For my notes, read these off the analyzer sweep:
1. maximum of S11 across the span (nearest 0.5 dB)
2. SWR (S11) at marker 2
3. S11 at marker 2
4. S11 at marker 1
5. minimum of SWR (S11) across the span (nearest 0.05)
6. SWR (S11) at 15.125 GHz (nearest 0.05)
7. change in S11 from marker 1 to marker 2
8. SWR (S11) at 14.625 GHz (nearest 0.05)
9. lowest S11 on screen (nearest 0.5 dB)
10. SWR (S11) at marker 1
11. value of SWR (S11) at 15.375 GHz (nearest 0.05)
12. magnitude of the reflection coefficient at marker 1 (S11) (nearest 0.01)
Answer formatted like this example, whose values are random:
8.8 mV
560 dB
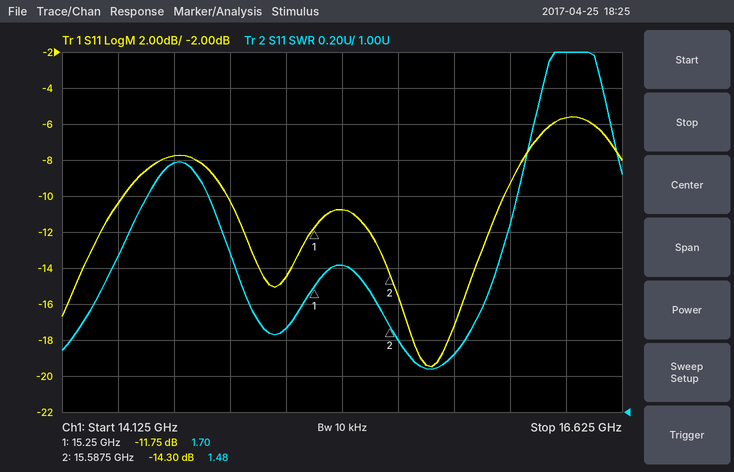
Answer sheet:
-5.5 dB
1.48
-14.30 dB
-11.75 dB
1.25
1.45
-2.55 dB
2.40
-19.5 dB
1.70
1.80
0.26
